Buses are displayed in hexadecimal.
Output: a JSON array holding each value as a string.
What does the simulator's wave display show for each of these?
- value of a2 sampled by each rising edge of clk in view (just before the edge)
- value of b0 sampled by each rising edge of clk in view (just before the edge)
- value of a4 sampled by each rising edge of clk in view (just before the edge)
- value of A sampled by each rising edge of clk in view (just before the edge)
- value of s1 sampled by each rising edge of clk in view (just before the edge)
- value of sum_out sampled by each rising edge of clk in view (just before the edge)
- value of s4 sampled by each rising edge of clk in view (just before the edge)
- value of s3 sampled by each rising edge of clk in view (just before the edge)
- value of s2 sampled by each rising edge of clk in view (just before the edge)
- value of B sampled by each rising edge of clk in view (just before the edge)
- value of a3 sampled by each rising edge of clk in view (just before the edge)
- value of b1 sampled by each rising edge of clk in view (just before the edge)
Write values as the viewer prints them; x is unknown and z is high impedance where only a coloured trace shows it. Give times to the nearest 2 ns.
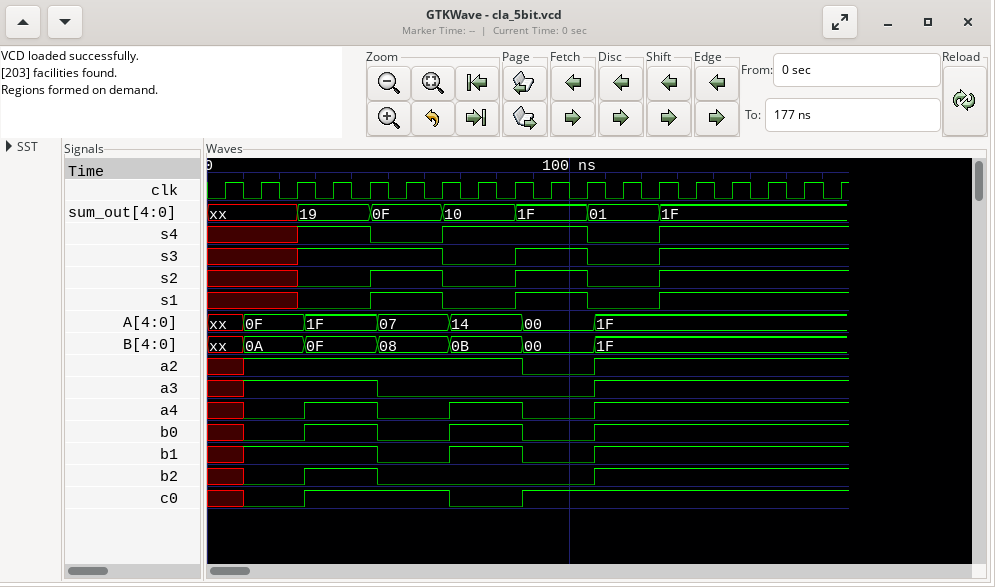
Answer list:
["x 1 1 1 1 1 1 1 1 0 0 1 1 1 1 1 1 1", "x 0 0 1 1 0 0 1 1 0 0 1 1 1 1 1 1 1", "x 0 0 1 1 0 0 1 1 0 0 1 1 1 1 1 1 1", "xx, 0F, 0F, 1F, 1F, 07, 07, 14, 14, 00, 00, 1F, 1F, 1F, 1F, 1F, 1F, 1F", "x x x 0 0 1 1 0 0 1 1 0 0 1 1 1 1 1", "xx, xx, xx, 19, 19, 0F, 0F, 10, 10, 1F, 1F, 01, 01, 1F, 1F, 1F, 1F, 1F", "x x x 1 1 0 0 1 1 1 1 0 0 1 1 1 1 1", "x x x 1 1 1 1 0 0 1 1 0 0 1 1 1 1 1", "x x x 0 0 1 1 0 0 1 1 0 0 1 1 1 1 1", "xx, 0A, 0A, 0F, 0F, 08, 08, 0B, 0B, 00, 00, 1F, 1F, 1F, 1F, 1F, 1F, 1F", "x 1 1 1 1 0 0 0 0 0 0 1 1 1 1 1 1 1", "x 1 1 1 1 0 0 1 1 0 0 1 1 1 1 1 1 1"]
